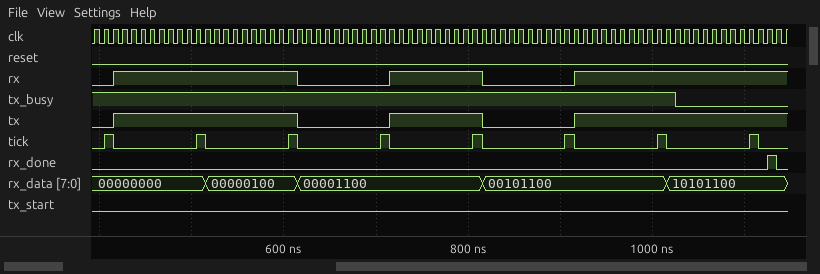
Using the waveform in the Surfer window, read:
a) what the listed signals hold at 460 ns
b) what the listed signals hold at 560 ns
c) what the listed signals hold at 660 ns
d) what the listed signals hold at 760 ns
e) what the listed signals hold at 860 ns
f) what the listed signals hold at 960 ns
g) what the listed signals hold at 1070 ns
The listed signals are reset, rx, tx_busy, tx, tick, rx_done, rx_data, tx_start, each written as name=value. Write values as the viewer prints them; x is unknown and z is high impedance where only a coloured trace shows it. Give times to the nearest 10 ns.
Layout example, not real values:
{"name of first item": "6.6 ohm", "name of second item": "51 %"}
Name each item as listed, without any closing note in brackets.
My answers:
{"what the listed signals hold at 460 ns": "reset=0, rx=1, tx_busy=1, tx=1, tick=0, rx_done=0, rx_data=00000000, tx_start=0", "what the listed signals hold at 560 ns": "reset=0, rx=1, tx_busy=1, tx=1, tick=0, rx_done=0, rx_data=00000100, tx_start=0", "what the listed signals hold at 660 ns": "reset=0, rx=0, tx_busy=1, tx=0, tick=0, rx_done=0, rx_data=00001100, tx_start=0", "what the listed signals hold at 760 ns": "reset=0, rx=1, tx_busy=1, tx=1, tick=0, rx_done=0, rx_data=00001100, tx_start=0", "what the listed signals hold at 860 ns": "reset=0, rx=0, tx_busy=1, tx=0, tick=0, rx_done=0, rx_data=00101100, tx_start=0", "what the listed signals hold at 960 ns": "reset=0, rx=1, tx_busy=1, tx=1, tick=0, rx_done=0, rx_data=00101100, tx_start=0", "what the listed signals hold at 1070 ns": "reset=0, rx=1, tx_busy=0, tx=1, tick=0, rx_done=0, rx_data=10101100, tx_start=0"}
